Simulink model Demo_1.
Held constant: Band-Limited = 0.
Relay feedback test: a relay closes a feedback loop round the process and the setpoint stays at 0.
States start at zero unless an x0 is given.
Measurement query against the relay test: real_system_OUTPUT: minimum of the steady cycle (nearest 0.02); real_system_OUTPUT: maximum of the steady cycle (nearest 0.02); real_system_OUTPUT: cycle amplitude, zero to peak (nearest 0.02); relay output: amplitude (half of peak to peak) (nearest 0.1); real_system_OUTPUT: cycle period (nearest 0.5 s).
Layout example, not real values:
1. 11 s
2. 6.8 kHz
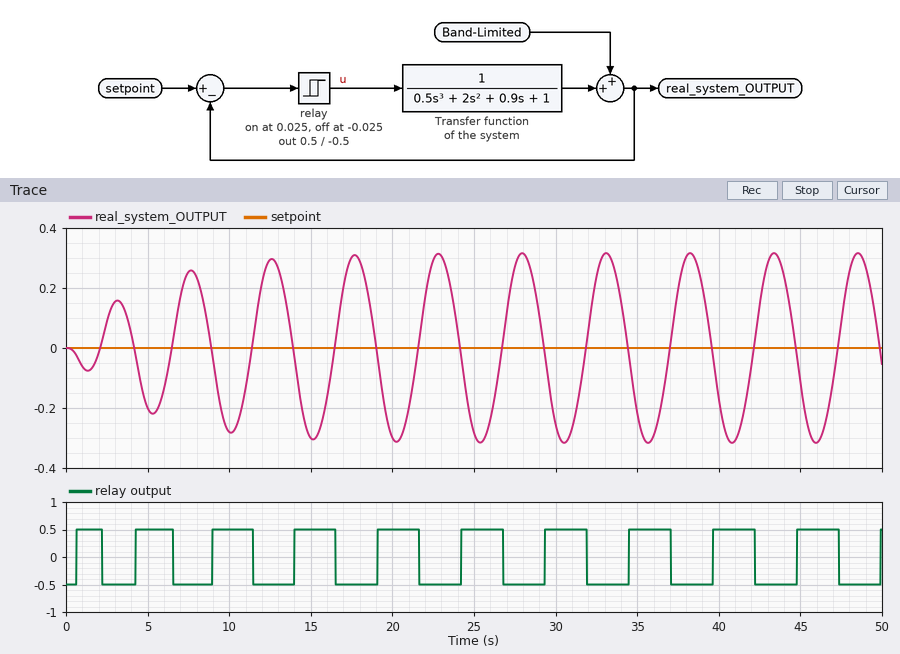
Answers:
1. -0.32
2. 0.32
3. 0.32
4. 0.5
5. 5.0 s
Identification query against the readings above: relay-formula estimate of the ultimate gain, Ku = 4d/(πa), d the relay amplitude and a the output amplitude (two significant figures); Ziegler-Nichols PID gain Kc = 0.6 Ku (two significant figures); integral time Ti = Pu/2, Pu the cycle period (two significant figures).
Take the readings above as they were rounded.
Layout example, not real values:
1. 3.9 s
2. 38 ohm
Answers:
1. 2.0
2. 1.2
3. 2.5 s
